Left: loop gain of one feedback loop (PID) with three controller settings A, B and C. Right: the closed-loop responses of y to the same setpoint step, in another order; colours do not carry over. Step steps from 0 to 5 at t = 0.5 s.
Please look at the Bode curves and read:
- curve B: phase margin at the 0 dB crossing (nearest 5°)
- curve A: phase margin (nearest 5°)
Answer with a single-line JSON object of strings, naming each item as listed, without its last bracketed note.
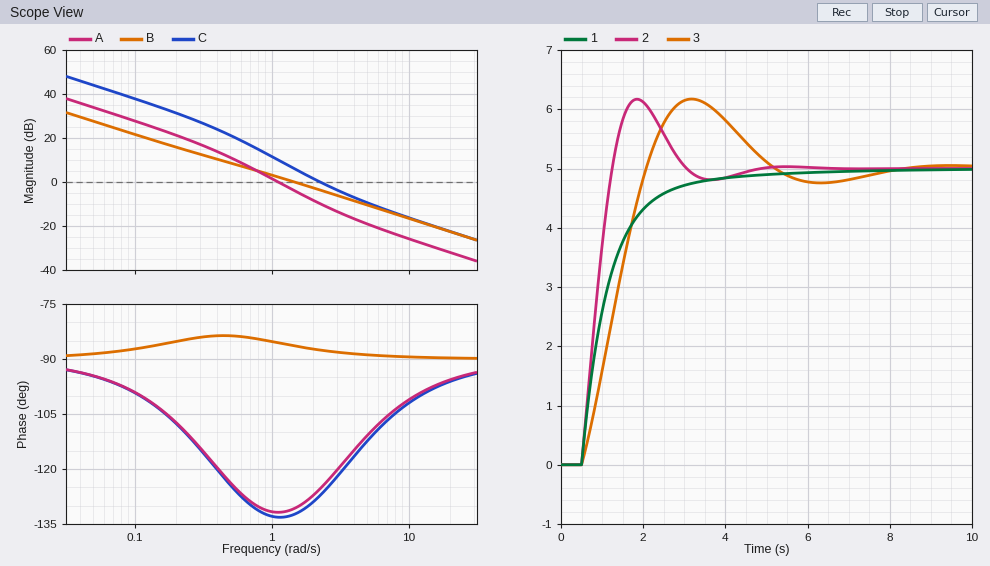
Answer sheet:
{"curve B: phase margin at the 0 dB crossing": "95°", "curve A: phase margin": "50°"}
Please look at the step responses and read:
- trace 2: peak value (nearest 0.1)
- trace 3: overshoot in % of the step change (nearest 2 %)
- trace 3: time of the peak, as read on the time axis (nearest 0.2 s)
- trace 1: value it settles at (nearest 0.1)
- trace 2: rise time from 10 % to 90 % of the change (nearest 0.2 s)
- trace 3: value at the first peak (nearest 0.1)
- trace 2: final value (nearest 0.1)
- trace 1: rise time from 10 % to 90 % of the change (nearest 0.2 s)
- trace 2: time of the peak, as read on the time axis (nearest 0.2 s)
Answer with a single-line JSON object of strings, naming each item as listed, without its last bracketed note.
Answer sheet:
{"trace 2: peak value": "6.2", "trace 3: overshoot in % of the step change": "24 %", "trace 3: time of the peak, as read on the time axis": "3.2 s", "trace 1: value it settles at": "5.0", "trace 2: rise time from 10 % to 90 % of the change": "0.6 s", "trace 3: value at the first peak": "6.2", "trace 2: final value": "5.0", "trace 1: rise time from 10 % to 90 % of the change": "1.8 s", "trace 2: time of the peak, as read on the time axis": "1.8 s"}
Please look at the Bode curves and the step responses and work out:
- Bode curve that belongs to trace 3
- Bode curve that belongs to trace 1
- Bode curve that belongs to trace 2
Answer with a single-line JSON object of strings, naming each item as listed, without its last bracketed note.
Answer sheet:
{"Bode curve that belongs to trace 3": "A", "Bode curve that belongs to trace 1": "B", "Bode curve that belongs to trace 2": "C"}
